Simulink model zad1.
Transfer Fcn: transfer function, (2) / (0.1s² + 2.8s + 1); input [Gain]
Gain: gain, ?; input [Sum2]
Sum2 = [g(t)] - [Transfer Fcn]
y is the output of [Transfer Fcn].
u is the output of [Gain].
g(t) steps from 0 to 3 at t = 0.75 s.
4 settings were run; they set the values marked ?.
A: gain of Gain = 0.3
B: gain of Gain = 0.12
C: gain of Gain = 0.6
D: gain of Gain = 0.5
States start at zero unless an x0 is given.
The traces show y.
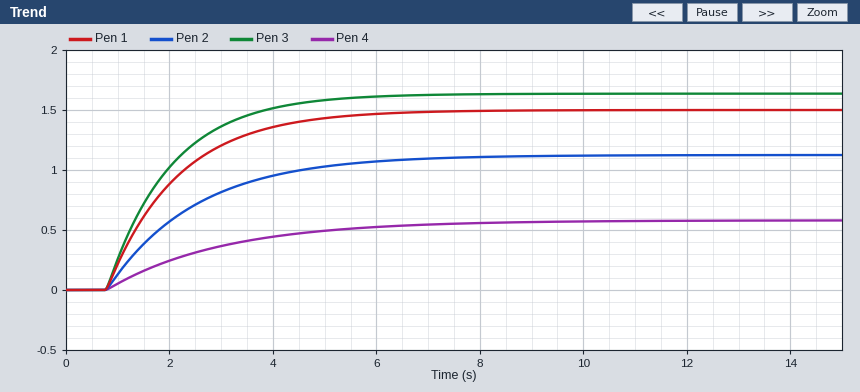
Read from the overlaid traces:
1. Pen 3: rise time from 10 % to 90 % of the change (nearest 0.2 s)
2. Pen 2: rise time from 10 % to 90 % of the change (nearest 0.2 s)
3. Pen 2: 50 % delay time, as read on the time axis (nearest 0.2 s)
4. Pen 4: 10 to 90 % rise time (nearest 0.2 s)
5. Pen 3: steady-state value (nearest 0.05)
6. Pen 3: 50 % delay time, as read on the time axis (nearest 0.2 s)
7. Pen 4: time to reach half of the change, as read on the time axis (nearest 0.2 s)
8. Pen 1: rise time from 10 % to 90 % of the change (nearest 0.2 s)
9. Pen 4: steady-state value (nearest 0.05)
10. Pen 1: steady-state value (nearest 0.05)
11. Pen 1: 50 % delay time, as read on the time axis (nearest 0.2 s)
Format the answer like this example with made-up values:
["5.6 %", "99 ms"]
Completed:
["2.8 s", "3.8 s", "2.0 s", "4.8 s", "1.65", "1.6 s", "2.4 s", "3.0 s", "0.60", "1.50", "1.8 s"]
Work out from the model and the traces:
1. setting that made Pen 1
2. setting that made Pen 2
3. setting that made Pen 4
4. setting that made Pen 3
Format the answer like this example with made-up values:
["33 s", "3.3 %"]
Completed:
["D", "A", "B", "C"]
